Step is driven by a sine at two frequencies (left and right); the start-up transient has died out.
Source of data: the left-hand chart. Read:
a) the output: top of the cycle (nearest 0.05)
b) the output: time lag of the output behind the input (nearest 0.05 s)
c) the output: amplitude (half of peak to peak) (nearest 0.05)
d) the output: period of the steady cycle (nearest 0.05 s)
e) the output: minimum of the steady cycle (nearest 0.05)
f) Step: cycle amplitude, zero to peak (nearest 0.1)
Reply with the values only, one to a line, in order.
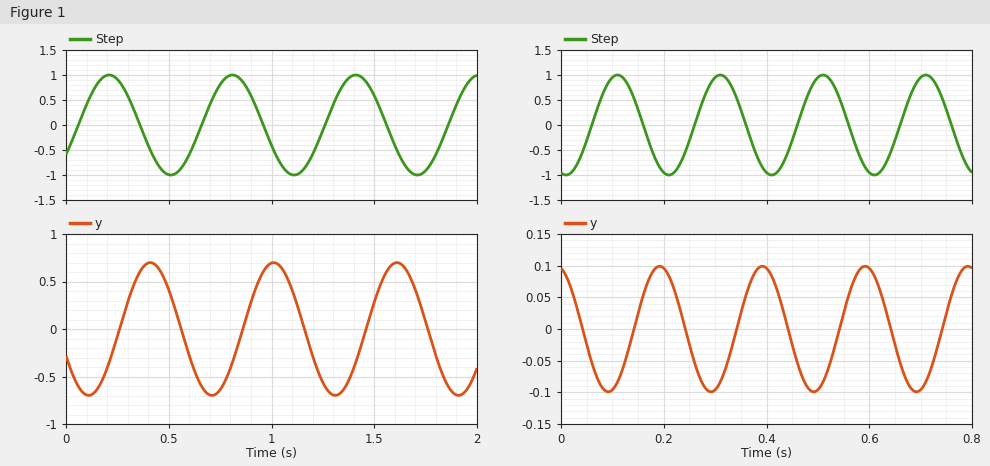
0.70
0.20 s
0.70
0.60 s
-0.70
1.0
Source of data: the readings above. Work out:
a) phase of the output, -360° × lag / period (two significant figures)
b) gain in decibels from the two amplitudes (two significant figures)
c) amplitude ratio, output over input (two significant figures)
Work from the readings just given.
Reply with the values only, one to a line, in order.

-120°
-3.1 dB
0.70
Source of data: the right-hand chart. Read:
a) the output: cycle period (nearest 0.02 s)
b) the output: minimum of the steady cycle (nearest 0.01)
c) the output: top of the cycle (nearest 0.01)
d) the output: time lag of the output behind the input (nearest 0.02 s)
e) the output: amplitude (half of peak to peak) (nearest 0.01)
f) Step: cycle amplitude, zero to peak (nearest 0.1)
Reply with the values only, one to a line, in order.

0.20 s
-0.10
0.10
0.08 s
0.10
1.0
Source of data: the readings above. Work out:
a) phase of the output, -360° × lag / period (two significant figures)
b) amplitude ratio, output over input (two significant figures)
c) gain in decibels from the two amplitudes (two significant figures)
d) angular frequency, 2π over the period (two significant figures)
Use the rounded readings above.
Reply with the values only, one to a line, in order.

-140°
0.10
-20 dB
31 rad/s
